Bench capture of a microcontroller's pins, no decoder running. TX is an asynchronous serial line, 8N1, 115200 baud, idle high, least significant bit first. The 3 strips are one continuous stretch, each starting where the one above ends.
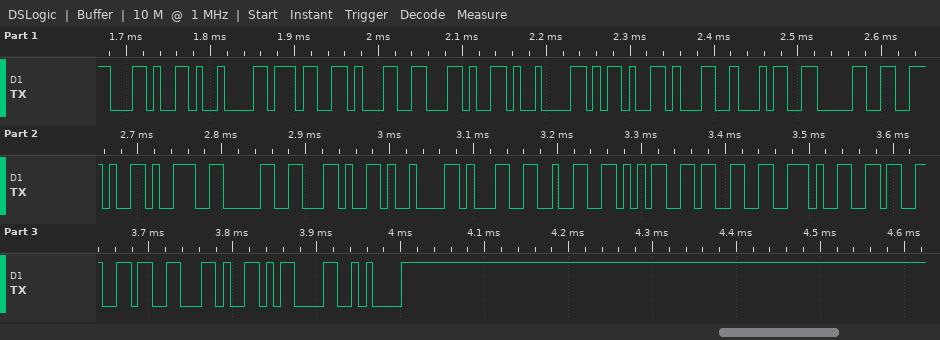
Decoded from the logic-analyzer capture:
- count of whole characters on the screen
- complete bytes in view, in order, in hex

25
2C 09 37 31 2C 09 2D 31 34 30 2E 39 30 2C 09 31 32 35 33 2E 36 36 2C 0D 0A
